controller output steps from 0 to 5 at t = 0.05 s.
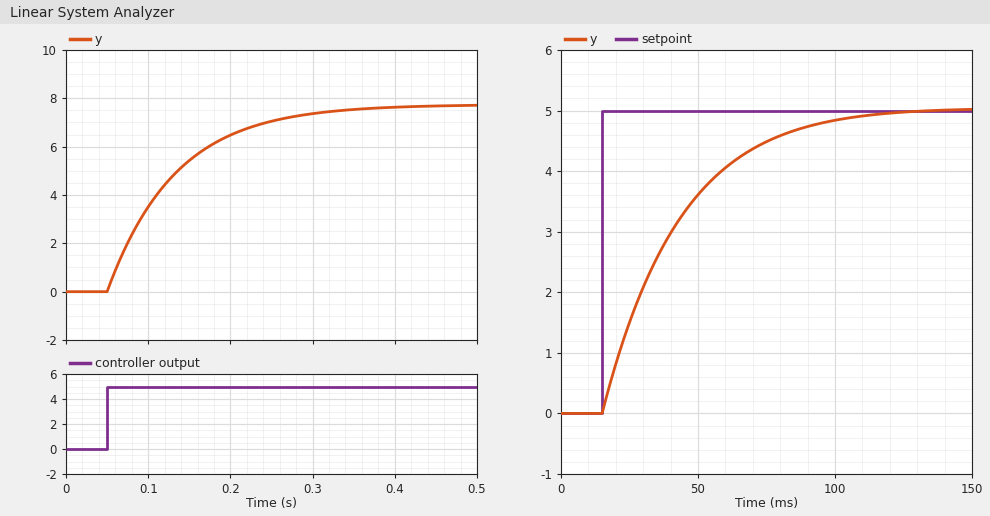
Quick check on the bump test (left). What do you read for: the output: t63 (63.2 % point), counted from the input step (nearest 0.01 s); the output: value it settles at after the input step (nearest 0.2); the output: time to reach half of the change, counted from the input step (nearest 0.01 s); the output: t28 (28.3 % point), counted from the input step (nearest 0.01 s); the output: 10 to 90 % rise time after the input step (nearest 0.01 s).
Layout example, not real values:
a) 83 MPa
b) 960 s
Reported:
a) 0.08 s
b) 7.8
c) 0.06 s
d) 0.03 s
e) 0.18 s
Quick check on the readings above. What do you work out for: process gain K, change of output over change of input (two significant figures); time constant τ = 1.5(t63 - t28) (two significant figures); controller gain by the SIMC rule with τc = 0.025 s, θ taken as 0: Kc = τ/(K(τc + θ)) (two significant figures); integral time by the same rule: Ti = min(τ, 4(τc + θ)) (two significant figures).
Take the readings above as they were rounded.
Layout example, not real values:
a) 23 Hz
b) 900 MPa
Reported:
a) 1.6
b) 0.075 s
c) 1.9
d) 0.075 s
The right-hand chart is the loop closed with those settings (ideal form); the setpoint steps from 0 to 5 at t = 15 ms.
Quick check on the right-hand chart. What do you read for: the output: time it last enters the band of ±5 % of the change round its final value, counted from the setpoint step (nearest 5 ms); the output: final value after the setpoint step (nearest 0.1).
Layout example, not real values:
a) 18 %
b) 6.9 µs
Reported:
a) 75 ms
b) 5.0
